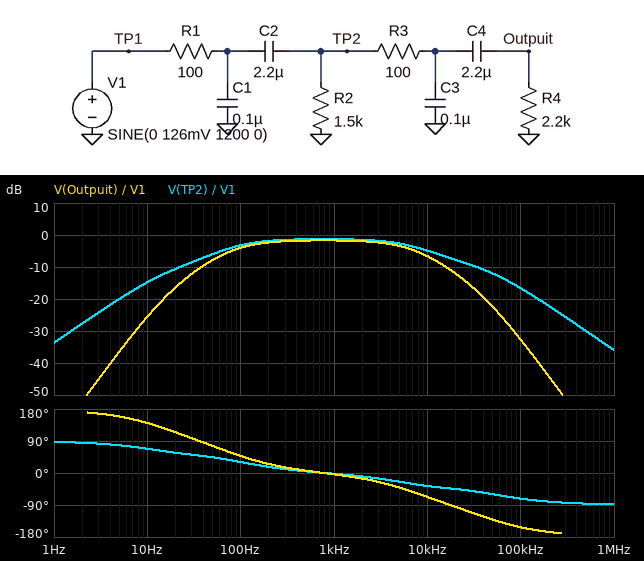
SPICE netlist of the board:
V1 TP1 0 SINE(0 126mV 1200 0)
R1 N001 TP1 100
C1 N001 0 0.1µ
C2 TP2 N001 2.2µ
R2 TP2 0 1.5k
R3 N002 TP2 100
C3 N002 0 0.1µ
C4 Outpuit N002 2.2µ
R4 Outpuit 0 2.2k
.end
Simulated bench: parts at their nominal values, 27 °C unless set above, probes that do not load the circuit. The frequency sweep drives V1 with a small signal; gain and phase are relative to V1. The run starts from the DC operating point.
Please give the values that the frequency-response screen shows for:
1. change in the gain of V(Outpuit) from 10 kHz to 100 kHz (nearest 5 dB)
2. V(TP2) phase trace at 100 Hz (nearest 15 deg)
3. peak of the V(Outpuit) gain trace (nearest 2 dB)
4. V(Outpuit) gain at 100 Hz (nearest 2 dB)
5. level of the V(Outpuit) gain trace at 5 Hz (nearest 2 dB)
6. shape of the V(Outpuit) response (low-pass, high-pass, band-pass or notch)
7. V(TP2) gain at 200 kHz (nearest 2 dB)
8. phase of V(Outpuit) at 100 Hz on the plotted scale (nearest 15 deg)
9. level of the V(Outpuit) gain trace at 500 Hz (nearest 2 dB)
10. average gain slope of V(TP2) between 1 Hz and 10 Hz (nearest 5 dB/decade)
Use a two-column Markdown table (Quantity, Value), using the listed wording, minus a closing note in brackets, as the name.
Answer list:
| Quantity | Value |
|---|---|
| change in the gain of V(Outpuit) from 10 kHz to 100 kHz | -25 dB |
| V(TP2) phase trace at 100 Hz | 30 deg |
| peak of the V(Outpuit) gain trace | -2 dB |
| V(Outpuit) gain at 100 Hz | -4 dB |
| level of the V(Outpuit) gain trace at 5 Hz | -36 dB |
| shape of the V(Outpuit) response | band-pass |
| V(TP2) gain at 200 kHz | -22 dB |
| phase of V(Outpuit) at 100 Hz on the plotted scale | 45 deg |
| level of the V(Outpuit) gain trace at 500 Hz | -2 dB |
| average gain slope of V(TP2) between 1 Hz and 10 Hz | 20 dB/decade |
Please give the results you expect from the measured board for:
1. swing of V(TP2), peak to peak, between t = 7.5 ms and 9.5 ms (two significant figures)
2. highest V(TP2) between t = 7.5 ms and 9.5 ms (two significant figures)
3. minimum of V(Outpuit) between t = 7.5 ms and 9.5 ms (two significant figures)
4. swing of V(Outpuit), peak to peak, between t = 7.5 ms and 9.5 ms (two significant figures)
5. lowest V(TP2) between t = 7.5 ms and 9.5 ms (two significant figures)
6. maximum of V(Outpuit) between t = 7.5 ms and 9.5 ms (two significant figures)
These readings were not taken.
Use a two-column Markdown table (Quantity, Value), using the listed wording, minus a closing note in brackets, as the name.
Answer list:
| Quantity | Value |
|---|---|
| swing of V(TP2), peak to peak, between t = 7.5 ms and 9.5 ms | 220 mV |
| highest V(TP2) between t = 7.5 ms and 9.5 ms | 110 mV |
| minimum of V(Outpuit) between t = 7.5 ms and 9.5 ms | -100 mV |
| swing of V(Outpuit), peak to peak, between t = 7.5 ms and 9.5 ms | 210 mV |
| lowest V(TP2) between t = 7.5 ms and 9.5 ms | -110 mV |
| maximum of V(Outpuit) between t = 7.5 ms and 9.5 ms | 100 mV |
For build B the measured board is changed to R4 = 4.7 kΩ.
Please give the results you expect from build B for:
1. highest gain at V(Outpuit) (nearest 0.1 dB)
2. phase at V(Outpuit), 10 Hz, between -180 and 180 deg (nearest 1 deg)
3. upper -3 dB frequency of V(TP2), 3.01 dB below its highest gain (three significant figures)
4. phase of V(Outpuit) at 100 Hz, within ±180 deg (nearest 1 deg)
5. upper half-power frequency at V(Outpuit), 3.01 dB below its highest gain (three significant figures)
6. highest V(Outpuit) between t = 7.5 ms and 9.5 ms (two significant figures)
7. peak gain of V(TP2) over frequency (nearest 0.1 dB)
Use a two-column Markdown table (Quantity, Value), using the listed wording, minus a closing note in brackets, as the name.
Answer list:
| Quantity | Value |
|---|---|
| highest gain at V(Outpuit) | -1.3 dB |
| phase at V(Outpuit), 10 Hz, between -180 and 180 deg | 127 deg |
| upper -3 dB frequency of V(TP2), 3.01 dB below its highest gain | 8.18 kHz |
| phase of V(Outpuit) at 100 Hz, within ±180 deg | 36 deg |
| upper half-power frequency at V(Outpuit), 3.01 dB below its highest gain | 6.73 kHz |
| highest V(Outpuit) between t = 7.5 ms and 9.5 ms | 110 mV |
| peak gain of V(TP2) over frequency | -1.1 dB |
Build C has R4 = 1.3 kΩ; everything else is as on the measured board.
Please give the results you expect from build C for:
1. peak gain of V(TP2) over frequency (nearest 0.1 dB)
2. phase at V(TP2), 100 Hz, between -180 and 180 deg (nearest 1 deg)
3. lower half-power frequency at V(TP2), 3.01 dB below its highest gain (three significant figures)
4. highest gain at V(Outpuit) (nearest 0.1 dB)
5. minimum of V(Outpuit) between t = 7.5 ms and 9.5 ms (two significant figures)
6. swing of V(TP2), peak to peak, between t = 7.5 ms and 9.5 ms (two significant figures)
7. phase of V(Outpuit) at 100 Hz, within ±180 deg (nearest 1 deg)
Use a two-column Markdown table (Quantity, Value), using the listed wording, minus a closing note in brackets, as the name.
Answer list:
| Quantity | Value |
|---|---|
| peak gain of V(TP2) over frequency | -1.5 dB |
| phase at V(TP2), 100 Hz, between -180 and 180 deg | 32 deg |
| lower half-power frequency at V(TP2), 3.01 dB below its highest gain | 91.2 Hz |
| highest gain at V(Outpuit) | -2.2 dB |
| minimum of V(Outpuit) between t = 7.5 ms and 9.5 ms | -98 mV |
| swing of V(TP2), peak to peak, between t = 7.5 ms and 9.5 ms | 210 mV |
| phase of V(Outpuit) at 100 Hz, within ±180 deg | 59 deg |
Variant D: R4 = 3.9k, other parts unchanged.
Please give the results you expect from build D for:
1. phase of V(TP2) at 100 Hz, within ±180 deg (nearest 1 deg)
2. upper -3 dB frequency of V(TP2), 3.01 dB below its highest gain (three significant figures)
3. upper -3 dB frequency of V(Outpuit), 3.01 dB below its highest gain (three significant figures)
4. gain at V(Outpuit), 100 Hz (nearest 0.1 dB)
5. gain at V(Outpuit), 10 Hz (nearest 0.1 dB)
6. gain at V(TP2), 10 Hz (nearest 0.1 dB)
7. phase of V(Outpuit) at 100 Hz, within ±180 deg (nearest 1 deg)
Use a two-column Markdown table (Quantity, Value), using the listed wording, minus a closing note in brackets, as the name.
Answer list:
| Quantity | Value |
|---|---|
| phase of V(TP2) at 100 Hz, within ±180 deg | 29 deg |
| upper -3 dB frequency of V(TP2), 3.01 dB below its highest gain | 8.25 kHz |
| upper -3 dB frequency of V(Outpuit), 3.01 dB below its highest gain | 6.79 kHz |
| gain at V(Outpuit), 100 Hz | -2.9 dB |
| gain at V(Outpuit), 10 Hz | -21.4 dB |
| gain at V(TP2), 10 Hz | -14.9 dB |
| phase of V(Outpuit) at 100 Hz, within ±180 deg | 39 deg |
